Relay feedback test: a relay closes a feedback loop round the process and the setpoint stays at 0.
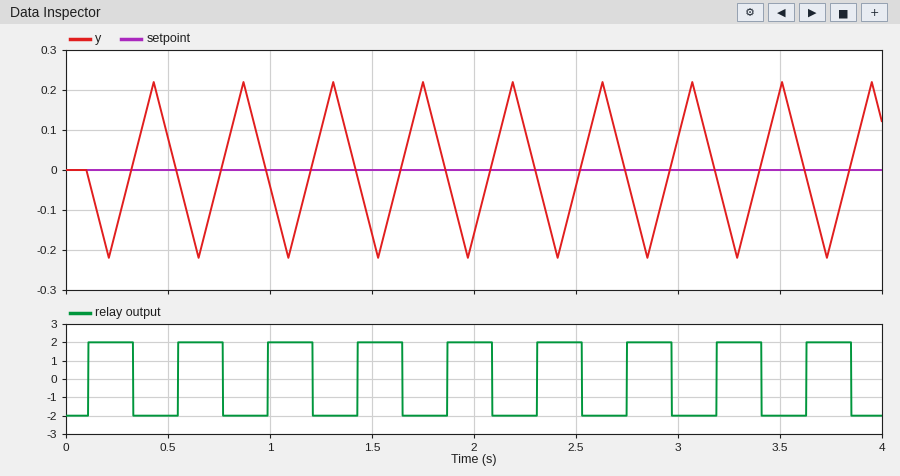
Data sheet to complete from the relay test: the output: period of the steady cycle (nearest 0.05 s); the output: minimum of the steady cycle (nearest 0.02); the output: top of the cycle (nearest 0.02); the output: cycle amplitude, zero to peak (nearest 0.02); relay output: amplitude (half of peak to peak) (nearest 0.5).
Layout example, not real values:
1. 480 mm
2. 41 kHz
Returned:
1. 0.45 s
2. -0.22
3. 0.22
4. 0.22
5. 2.0
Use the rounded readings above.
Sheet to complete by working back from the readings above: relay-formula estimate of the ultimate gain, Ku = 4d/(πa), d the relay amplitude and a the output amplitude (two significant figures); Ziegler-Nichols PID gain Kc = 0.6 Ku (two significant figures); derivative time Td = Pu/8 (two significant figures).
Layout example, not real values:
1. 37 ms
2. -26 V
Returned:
1. 12
2. 7.2
3. 0.056 s
